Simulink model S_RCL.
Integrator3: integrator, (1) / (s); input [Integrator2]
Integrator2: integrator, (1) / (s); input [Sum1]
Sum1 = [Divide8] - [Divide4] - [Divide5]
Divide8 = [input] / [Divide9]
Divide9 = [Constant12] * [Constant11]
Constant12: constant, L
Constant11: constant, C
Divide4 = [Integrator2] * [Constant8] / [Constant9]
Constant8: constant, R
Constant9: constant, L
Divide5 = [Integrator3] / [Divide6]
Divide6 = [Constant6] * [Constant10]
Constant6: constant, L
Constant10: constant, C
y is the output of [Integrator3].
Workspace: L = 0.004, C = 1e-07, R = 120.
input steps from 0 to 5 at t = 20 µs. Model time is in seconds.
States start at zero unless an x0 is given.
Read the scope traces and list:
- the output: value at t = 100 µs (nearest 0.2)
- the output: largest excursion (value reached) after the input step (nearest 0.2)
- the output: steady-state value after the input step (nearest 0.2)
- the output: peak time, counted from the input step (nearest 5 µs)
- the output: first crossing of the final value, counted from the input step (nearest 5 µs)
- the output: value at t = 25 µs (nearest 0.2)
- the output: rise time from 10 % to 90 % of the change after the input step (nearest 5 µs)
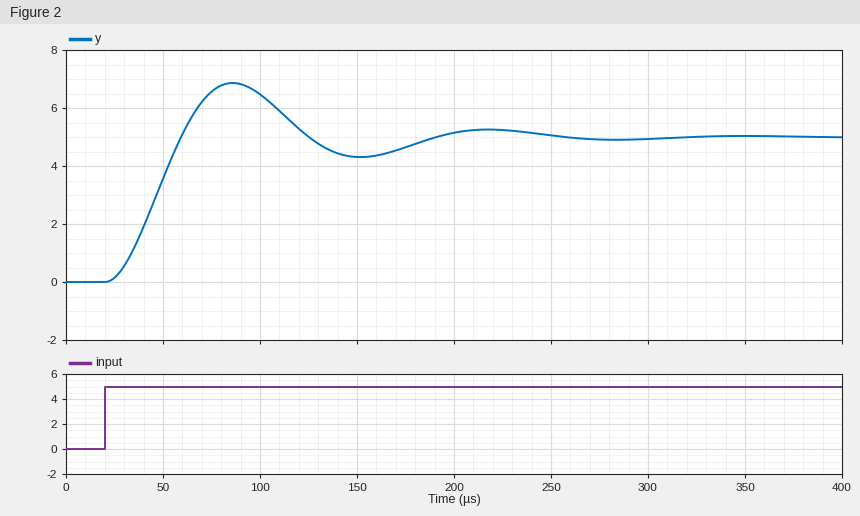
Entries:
6.4
6.8
5.0
65 µs
40 µs
0.2
25 µs
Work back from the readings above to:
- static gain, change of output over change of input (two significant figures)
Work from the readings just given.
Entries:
1.0
